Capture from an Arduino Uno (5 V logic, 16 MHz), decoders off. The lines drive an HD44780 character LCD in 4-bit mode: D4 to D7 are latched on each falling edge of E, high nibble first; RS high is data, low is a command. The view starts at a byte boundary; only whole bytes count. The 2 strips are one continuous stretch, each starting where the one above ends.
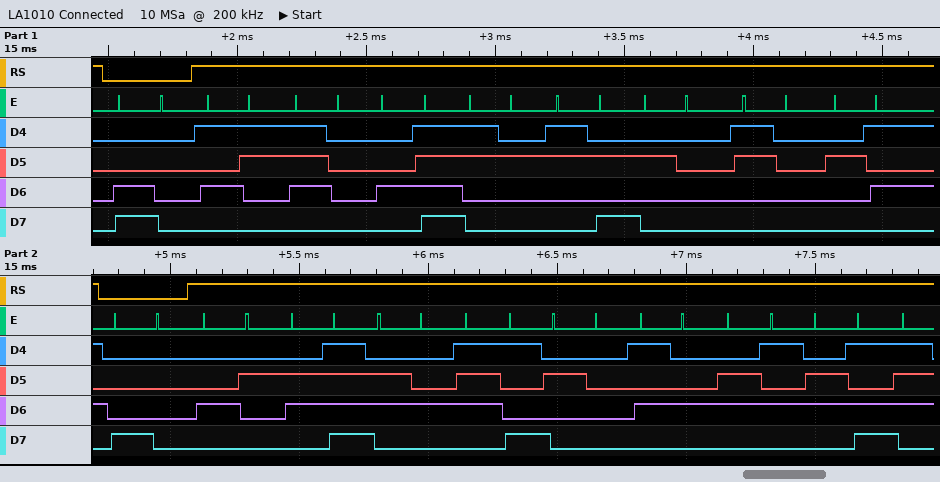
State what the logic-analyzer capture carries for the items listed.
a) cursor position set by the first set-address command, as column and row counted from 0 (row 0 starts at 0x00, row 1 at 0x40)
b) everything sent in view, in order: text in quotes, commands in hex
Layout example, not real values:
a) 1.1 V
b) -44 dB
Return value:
a) column 0, row 1
b) 0xC0 "SpO2: 0%" 0x80 "Body Tem"
